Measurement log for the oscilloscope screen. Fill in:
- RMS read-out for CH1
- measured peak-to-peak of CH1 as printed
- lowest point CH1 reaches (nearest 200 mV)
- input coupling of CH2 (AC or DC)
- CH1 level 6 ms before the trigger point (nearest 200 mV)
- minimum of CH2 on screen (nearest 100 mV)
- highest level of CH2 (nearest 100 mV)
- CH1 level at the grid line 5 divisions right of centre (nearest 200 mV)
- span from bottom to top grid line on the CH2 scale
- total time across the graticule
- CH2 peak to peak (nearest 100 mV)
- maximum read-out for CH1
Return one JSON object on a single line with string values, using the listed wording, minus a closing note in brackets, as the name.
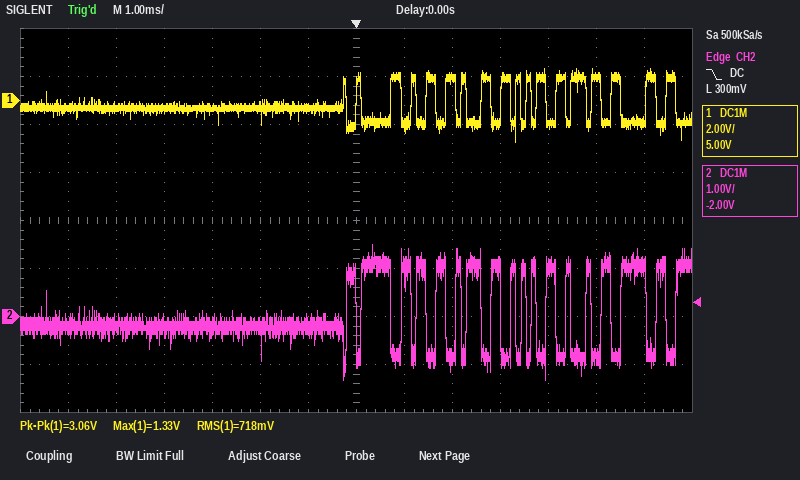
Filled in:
{"RMS read-out for CH1": "718 mV", "measured peak-to-peak of CH1 as printed": "3.06 V", "lowest point CH1 reaches": "-1.8 V", "input coupling of CH2": "DC", "CH1 level 6 ms before the trigger point": "-200 mV", "minimum of CH2 on screen": "-1.3 V", "highest level of CH2": "1.5 V", "CH1 level at the grid line 5 divisions right of centre": "1.0 V", "span from bottom to top grid line on the CH2 scale": "8 V", "total time across the graticule": "14 ms", "CH2 peak to peak": "2.8 V", "maximum read-out for CH1": "1.33 V"}
